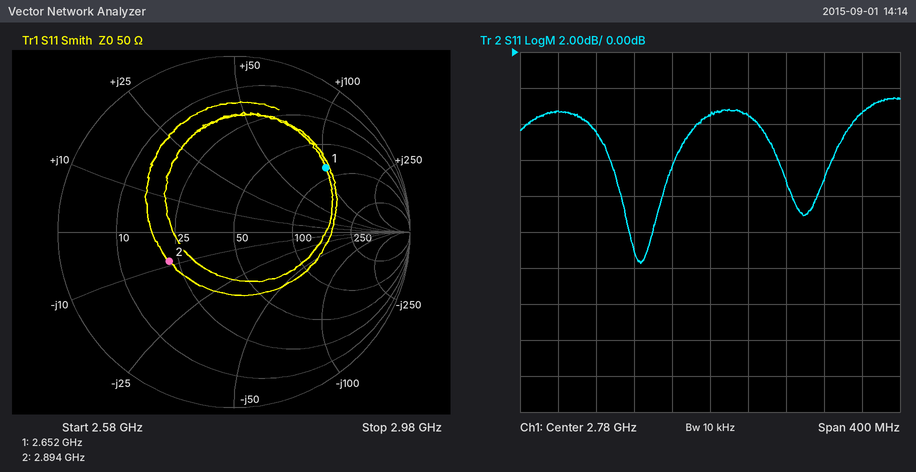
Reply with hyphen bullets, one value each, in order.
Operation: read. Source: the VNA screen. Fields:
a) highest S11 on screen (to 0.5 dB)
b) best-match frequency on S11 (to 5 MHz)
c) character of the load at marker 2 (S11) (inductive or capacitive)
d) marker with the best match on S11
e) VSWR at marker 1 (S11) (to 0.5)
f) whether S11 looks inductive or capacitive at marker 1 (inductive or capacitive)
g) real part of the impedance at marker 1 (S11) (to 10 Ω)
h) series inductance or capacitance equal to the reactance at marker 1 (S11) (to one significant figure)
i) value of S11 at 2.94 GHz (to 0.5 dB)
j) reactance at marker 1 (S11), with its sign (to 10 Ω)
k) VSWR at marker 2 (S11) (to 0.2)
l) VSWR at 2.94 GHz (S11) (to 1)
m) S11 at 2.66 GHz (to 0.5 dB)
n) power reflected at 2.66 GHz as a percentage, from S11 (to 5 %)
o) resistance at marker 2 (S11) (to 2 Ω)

- -2.5 dB
- 2.705 GHz
- capacitive
- marker 2
- 4.5
- inductive
- 80 Ω
- 6 nH
- -3.5 dB
- +100 Ω
- 2.4
- 5
- -4.5 dB
- 35 %
- 22 Ω
